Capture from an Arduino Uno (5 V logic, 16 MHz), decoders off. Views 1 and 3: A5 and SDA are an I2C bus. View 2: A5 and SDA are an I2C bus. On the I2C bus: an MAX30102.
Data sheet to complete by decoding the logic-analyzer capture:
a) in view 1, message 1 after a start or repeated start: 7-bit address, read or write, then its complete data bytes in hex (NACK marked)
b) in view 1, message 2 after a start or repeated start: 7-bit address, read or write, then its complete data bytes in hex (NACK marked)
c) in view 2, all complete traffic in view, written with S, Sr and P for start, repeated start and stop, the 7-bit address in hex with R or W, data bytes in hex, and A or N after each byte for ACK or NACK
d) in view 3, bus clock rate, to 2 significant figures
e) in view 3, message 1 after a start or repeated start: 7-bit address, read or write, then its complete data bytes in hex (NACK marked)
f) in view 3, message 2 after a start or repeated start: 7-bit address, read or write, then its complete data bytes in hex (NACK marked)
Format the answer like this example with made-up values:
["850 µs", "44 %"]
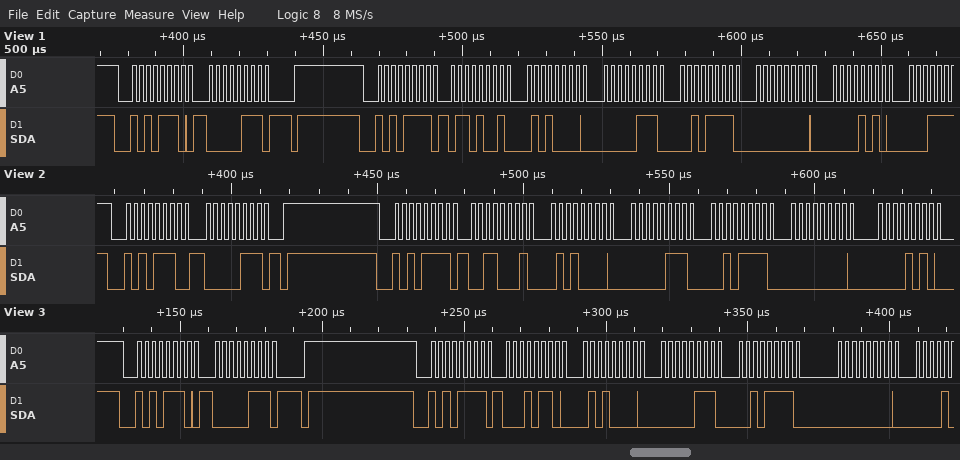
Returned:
["0x57 write: 07", "0x57 read: 69 50 07 2F 00 0A", "S 57W A 07 A P S 57R A 31 A 50 A 07 A 2F A 00 A 0A A", "400 kHz", "0x57 write: 07", "0x57 read: 16 50 07 2F 00"]
